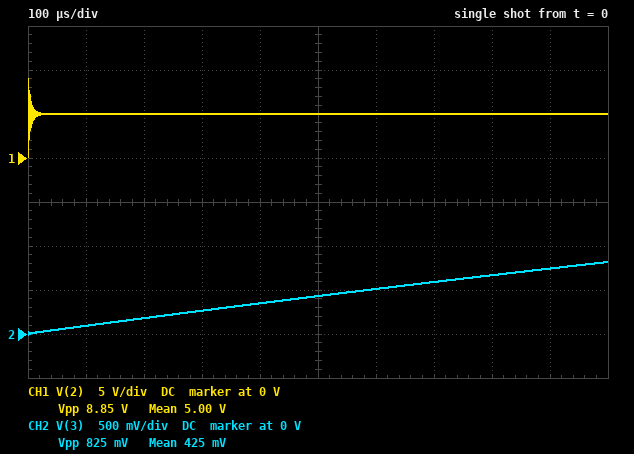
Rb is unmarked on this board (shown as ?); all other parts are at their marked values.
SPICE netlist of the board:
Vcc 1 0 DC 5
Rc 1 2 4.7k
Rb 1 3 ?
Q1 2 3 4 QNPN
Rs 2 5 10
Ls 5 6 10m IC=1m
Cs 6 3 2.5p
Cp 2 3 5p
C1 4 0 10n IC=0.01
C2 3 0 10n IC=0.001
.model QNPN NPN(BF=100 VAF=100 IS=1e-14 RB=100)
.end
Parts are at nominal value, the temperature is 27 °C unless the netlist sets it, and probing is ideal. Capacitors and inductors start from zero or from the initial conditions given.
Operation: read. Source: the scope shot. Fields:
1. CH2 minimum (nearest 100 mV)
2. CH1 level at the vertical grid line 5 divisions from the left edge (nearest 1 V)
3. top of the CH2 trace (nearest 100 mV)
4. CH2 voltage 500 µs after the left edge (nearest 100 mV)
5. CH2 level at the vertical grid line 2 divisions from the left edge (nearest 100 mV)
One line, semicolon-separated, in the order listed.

0 V; 5 V; 800 mV; 400 mV; 200 mV
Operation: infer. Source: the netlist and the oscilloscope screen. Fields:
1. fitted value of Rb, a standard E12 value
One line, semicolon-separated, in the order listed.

560 kΩ
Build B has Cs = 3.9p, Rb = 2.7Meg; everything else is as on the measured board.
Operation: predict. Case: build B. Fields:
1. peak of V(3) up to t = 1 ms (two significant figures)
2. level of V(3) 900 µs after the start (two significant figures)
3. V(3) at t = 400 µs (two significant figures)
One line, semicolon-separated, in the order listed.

190 mV; 170 mV; 79 mV
